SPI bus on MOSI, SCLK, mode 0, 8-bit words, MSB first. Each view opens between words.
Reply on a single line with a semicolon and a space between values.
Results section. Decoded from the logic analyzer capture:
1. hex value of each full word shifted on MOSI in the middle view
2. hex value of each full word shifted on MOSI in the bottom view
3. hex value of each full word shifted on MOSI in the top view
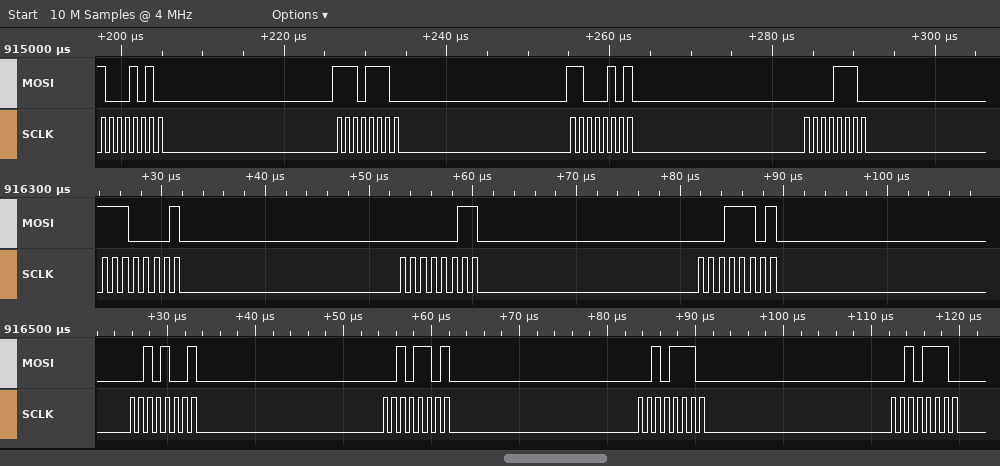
E1, 03, 1D; 29, 2D, 2E, 2E; 8A, EE, C5, 0E
